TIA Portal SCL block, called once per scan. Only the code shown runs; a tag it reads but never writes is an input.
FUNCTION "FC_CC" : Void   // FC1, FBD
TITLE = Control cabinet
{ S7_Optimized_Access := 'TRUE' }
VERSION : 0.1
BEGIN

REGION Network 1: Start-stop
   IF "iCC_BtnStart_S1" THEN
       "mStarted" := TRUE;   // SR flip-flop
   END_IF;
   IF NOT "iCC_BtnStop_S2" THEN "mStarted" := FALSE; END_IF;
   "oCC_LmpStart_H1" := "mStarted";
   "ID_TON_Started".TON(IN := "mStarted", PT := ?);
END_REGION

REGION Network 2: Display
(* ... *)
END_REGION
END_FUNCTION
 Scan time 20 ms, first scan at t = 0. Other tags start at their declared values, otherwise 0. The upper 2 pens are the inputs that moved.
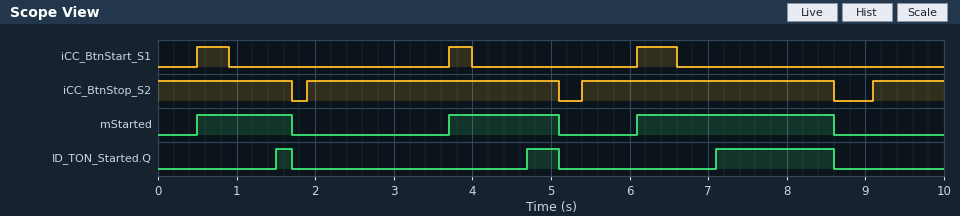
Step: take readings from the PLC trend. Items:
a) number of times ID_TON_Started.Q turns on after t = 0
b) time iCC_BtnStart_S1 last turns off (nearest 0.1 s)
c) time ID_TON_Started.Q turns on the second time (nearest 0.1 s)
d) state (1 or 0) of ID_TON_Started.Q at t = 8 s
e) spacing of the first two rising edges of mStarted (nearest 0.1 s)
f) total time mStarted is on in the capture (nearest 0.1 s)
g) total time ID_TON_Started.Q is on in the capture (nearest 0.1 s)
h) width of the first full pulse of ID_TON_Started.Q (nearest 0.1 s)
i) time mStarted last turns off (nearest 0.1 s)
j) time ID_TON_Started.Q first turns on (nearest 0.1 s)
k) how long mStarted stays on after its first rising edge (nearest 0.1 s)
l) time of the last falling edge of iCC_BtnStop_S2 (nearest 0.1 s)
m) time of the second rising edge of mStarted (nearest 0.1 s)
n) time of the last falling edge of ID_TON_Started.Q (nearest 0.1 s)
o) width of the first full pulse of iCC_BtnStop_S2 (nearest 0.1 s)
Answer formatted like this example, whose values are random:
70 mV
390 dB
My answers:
3
6.6 s
4.7 s
1
3.2 s
5.1 s
2.1 s
0.2 s
8.6 s
1.5 s
1.2 s
8.6 s
3.7 s
8.6 s
3.2 s
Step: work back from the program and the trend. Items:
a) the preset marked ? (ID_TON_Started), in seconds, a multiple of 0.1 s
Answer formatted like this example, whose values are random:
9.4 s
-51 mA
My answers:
1.0 s
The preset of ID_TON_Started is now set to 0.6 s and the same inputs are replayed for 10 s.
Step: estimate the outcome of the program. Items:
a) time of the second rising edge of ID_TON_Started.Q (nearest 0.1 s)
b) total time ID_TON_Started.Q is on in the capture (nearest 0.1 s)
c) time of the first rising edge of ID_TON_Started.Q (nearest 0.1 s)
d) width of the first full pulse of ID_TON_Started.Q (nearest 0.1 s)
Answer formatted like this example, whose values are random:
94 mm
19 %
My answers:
4.3 s
3.3 s
1.1 s
0.6 s
